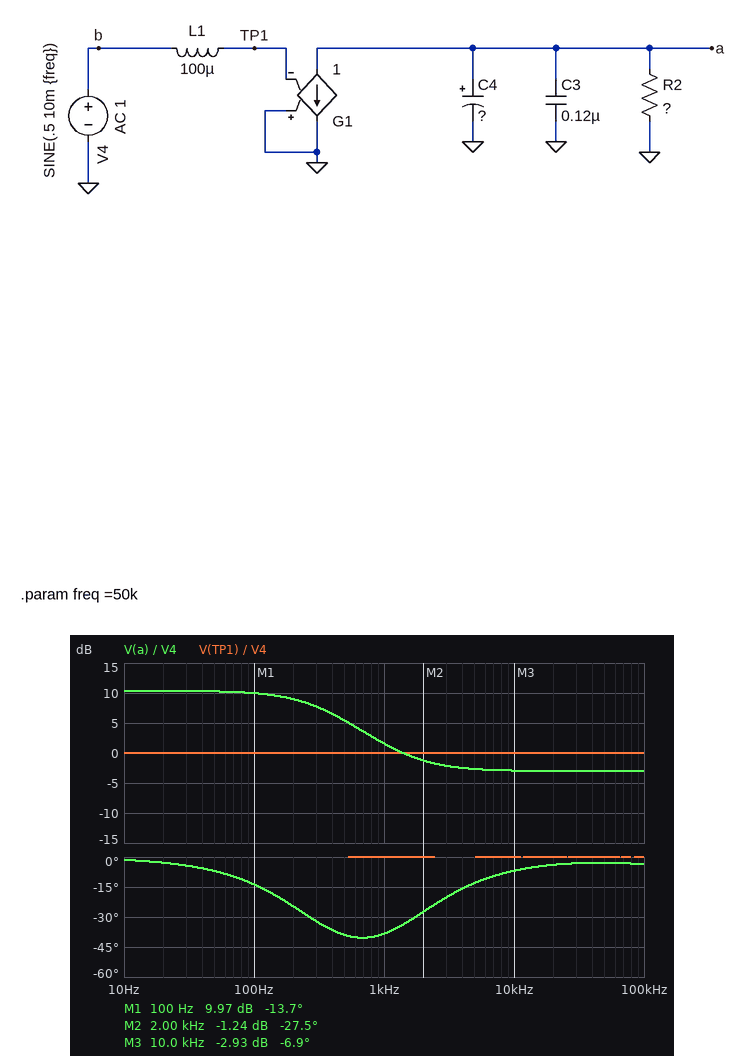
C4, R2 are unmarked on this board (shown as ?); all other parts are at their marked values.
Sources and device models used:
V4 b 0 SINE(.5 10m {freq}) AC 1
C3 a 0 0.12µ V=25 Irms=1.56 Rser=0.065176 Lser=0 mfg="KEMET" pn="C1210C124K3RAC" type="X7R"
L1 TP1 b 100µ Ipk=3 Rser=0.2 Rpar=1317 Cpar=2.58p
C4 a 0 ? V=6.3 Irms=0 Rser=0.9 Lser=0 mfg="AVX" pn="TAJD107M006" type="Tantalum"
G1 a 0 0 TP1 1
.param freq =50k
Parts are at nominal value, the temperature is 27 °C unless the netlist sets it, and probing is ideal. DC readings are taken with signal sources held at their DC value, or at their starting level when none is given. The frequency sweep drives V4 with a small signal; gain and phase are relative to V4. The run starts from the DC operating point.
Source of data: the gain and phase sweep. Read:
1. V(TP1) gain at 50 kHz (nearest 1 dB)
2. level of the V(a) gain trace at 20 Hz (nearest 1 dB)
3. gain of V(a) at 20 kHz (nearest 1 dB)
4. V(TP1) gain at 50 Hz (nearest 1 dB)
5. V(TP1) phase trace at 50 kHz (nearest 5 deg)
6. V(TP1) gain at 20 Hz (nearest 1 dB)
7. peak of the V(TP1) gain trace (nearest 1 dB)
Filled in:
0 dB
10 dB
-3 dB
0 dB
0 deg
0 dB
0 dB
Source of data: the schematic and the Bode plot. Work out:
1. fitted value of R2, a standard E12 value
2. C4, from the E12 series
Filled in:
3.3 Ω
120 µF
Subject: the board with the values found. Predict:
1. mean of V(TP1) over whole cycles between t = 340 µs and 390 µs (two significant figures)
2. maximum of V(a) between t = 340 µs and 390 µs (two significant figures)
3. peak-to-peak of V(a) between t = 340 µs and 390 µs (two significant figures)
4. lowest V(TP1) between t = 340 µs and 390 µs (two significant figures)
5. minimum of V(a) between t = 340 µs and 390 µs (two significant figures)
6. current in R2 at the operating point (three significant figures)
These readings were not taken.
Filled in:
500 mV
1.7 V
14 mV
490 mV
1.6 V
500 mA
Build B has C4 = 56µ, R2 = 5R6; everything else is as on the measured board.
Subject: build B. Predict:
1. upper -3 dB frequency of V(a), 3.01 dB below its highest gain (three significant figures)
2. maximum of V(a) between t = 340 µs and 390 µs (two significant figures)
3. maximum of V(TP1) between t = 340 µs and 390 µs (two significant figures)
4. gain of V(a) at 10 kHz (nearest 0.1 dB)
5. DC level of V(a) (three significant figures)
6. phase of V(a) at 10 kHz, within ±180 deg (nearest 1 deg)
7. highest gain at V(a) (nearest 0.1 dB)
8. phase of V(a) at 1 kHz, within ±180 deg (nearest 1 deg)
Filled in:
445 Hz
2.8 V
510 mV
-1.8 dB
2.80 V
-15 deg
15.0 dB
-49 deg
